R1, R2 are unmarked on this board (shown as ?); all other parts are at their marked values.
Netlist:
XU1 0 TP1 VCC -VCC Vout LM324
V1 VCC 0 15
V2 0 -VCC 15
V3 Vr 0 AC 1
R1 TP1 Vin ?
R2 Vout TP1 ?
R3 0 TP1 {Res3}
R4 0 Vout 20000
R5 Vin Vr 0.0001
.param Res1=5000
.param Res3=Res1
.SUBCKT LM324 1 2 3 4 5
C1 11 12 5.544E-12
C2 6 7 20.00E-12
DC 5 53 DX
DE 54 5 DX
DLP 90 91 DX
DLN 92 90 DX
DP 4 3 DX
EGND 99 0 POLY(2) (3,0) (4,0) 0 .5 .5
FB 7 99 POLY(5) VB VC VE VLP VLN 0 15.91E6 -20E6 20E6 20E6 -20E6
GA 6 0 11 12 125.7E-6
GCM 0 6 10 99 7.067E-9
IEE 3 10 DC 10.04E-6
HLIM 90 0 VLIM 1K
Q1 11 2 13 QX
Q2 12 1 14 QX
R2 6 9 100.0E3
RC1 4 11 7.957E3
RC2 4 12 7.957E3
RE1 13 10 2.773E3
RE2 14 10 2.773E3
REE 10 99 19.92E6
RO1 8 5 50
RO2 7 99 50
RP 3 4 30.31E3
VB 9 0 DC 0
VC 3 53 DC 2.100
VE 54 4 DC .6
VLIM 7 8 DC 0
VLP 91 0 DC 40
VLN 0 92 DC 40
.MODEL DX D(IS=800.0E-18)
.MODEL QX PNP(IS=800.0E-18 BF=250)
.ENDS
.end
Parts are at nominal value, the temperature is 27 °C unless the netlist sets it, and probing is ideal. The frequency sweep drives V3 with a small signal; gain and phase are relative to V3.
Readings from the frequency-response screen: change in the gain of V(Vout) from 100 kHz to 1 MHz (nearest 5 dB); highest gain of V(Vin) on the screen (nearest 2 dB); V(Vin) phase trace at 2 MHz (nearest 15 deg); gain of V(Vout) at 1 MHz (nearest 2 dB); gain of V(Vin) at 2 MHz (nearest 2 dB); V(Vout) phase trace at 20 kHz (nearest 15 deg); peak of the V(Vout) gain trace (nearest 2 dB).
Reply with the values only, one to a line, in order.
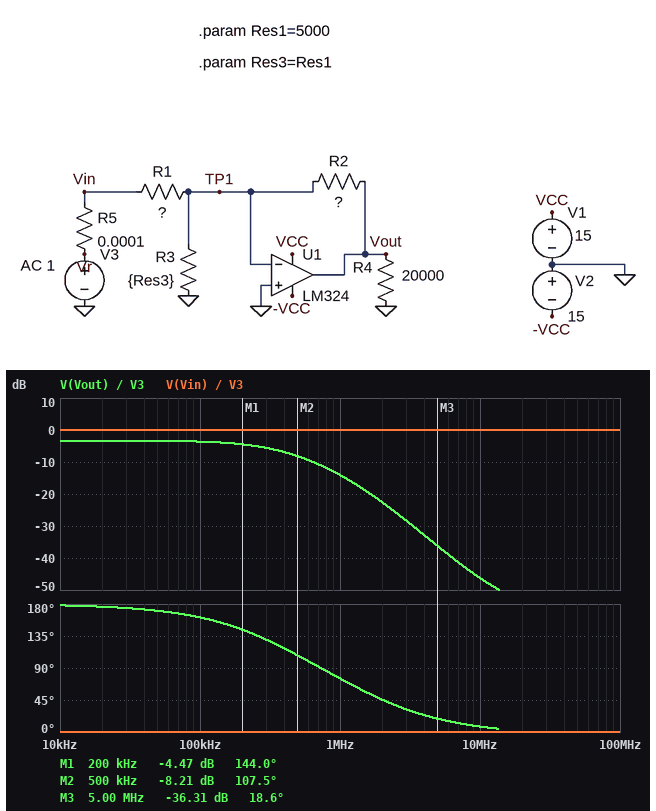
-10 dB
0 dB
0 deg
-14 dB
0 dB
180 deg
-4 dB
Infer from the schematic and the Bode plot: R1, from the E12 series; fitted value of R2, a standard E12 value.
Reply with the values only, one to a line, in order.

12 kΩ
8.2 kΩ
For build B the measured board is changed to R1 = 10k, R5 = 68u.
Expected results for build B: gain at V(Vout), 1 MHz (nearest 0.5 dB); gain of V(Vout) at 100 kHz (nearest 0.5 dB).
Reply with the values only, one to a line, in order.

-13.0 dB
-2.0 dB
